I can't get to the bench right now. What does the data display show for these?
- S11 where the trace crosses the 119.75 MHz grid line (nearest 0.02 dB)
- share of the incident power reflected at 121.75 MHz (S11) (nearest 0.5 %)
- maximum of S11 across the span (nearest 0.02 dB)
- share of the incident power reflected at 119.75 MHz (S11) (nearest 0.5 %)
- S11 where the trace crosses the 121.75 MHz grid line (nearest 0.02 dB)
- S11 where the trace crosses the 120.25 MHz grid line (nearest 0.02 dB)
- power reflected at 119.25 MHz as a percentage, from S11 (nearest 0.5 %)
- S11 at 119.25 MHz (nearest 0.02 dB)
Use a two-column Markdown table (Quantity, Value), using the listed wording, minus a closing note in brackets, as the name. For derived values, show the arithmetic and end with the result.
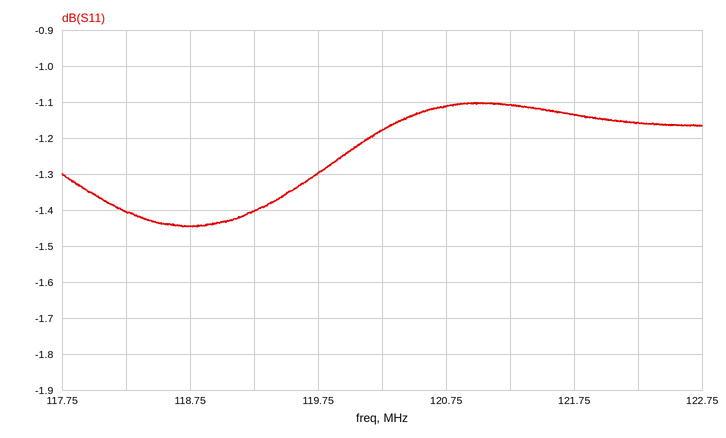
| Quantity | Value |
|---|---|
| S11 where the trace crosses the 119.75 MHz grid line | -1.30 dB |
| share of the incident power reflected at 121.75 MHz (S11) | 10^(-1.14/10) ≈ 76.9 %, so 77.0 % to the nearest 0.5 % |
| maximum of S11 across the span | -1.10 dB |
| share of the incident power reflected at 119.75 MHz (S11) | 10^(-1.3/10) ≈ 74.1 %, so 74.0 % to the nearest 0.5 % |
| S11 where the trace crosses the 121.75 MHz grid line | -1.14 dB |
| S11 where the trace crosses the 120.25 MHz grid line | -1.18 dB |
| power reflected at 119.25 MHz as a percentage, from S11 | 10^(-1.4/10) ≈ 72.4 %, so 72.5 % to the nearest 0.5 % |
| S11 at 119.25 MHz | -1.40 dB |
